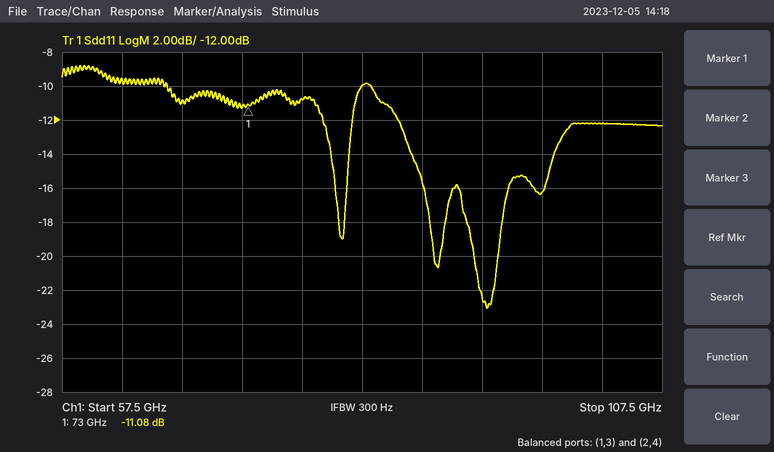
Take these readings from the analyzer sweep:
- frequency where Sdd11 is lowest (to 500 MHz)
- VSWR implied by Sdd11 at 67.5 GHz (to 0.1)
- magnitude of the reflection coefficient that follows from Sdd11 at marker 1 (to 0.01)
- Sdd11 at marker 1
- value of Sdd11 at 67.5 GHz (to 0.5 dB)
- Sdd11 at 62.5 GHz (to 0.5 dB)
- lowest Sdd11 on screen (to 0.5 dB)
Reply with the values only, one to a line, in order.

93.0 GHz
1.8
0.28
-11.08 dB
-11.0 dB
-9.5 dB
-23.0 dB
